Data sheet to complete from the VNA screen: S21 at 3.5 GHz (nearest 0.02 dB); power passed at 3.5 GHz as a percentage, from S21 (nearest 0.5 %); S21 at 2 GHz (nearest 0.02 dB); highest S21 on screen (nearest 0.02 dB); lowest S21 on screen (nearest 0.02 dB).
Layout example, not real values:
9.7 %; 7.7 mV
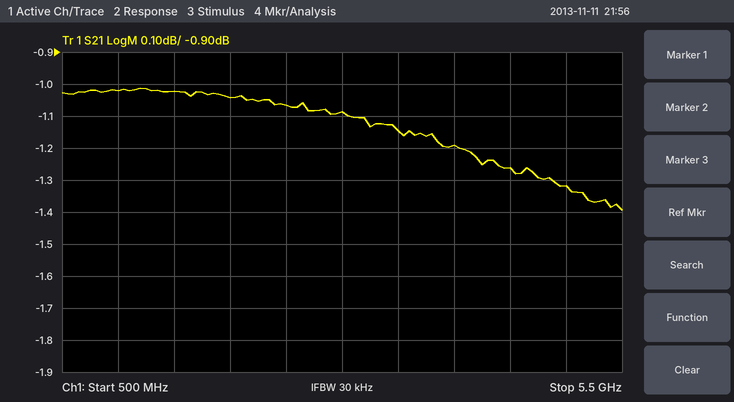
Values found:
-1.14 dB; 77.0 %; -1.04 dB; -1.02 dB; -1.40 dB
